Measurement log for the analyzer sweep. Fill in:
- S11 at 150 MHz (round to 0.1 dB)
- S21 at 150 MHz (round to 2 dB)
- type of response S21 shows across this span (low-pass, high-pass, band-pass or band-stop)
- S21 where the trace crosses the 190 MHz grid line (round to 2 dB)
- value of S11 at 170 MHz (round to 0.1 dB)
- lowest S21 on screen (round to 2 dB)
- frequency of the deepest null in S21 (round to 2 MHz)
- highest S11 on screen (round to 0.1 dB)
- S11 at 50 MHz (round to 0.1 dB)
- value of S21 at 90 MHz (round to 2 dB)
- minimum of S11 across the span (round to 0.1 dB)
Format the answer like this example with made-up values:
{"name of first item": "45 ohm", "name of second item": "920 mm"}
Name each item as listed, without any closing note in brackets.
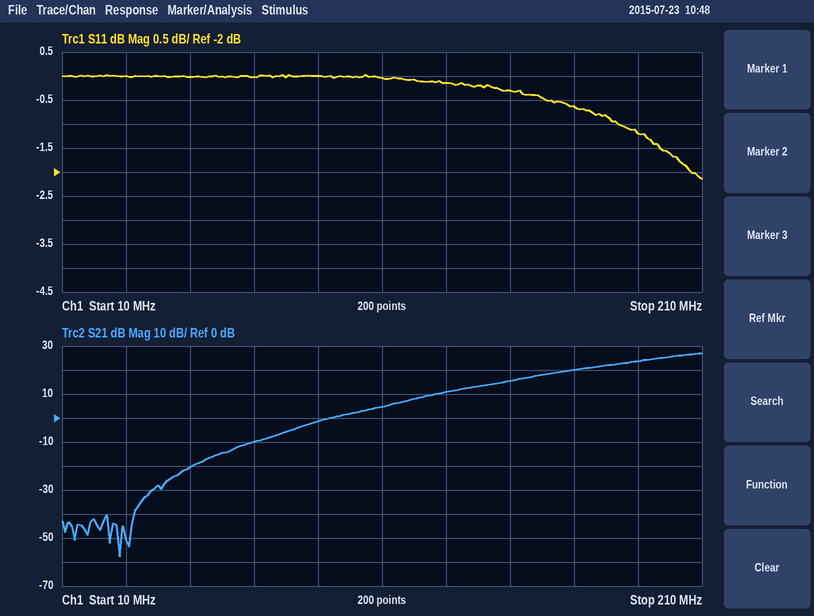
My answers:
{"S11 at 150 MHz": "-0.3 dB", "S21 at 150 MHz": "16 dB", "type of response S21 shows across this span": "high-pass", "S21 where the trace crosses the 190 MHz grid line": "24 dB", "value of S11 at 170 MHz": "-0.6 dB", "lowest S21 on screen": "-58 dB", "frequency of the deepest null in S21": "28 MHz", "highest S11 on screen": "0.0 dB", "S11 at 50 MHz": "0.0 dB", "value of S21 at 90 MHz": "-2 dB", "minimum of S11 across the span": "-2.1 dB"}
